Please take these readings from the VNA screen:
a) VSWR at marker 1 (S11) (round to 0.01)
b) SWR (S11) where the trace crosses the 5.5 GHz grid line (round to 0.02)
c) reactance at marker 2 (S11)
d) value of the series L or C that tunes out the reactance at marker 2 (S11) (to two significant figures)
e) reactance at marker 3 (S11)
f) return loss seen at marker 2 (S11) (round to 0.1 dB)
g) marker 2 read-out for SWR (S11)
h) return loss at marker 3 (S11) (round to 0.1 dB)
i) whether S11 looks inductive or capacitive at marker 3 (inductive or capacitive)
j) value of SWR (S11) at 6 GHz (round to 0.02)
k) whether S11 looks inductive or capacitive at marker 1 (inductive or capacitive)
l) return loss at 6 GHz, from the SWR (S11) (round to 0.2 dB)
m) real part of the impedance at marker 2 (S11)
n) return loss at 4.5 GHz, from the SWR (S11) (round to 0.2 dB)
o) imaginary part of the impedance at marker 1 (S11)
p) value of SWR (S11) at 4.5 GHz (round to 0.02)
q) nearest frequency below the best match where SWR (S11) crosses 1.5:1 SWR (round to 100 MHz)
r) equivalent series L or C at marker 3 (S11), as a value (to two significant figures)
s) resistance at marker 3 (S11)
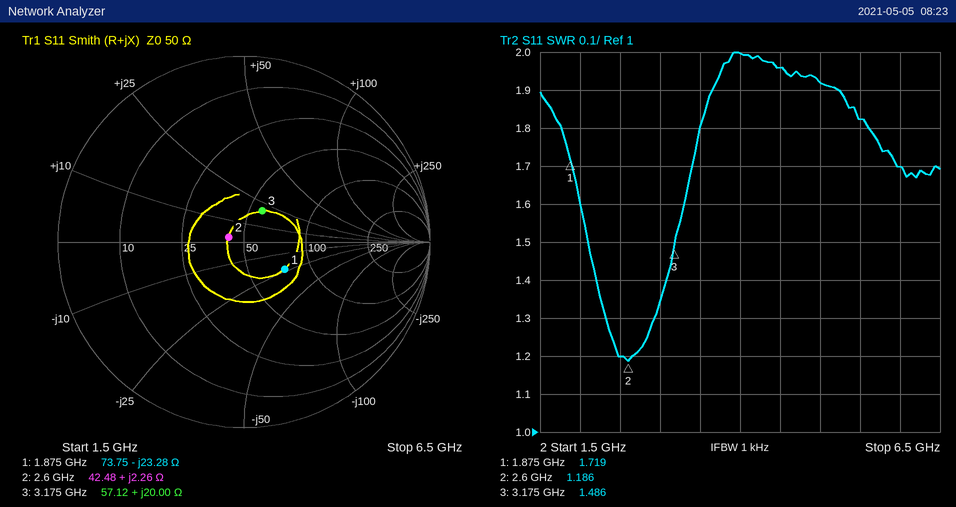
1.72
1.82
+2.26 Ω
27 pF
+20.00 Ω
21.4 dB
1.186
14.2 dB
inductive
1.70
capacitive
11.8 dB
42.48 Ω
9.8 dB
-23.28 Ω
1.96
2.1 GHz
1.0 nH
57.12 Ω
